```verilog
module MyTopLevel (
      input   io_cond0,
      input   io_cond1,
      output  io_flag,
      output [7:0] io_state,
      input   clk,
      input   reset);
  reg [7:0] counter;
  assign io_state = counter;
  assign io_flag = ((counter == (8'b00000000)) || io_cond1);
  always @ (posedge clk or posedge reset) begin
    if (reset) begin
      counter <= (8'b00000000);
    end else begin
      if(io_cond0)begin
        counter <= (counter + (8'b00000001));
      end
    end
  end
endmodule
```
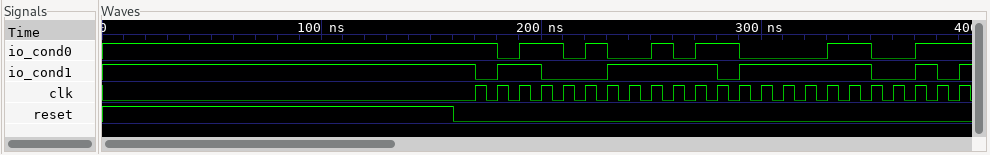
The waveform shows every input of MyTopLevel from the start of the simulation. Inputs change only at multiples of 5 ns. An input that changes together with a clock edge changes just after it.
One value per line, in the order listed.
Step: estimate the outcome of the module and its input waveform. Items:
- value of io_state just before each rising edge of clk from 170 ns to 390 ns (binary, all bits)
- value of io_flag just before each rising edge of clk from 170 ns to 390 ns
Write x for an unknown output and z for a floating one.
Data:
00000000, 00000001, 00000010, 00000010, 00000011, 00000100, 00000100, 00000101, 00000101, 00000101, 00000110, 00000110, 00000111, 00001000, 00001000, 00001000, 00001000, 00001000, 00001001, 00001010, 00001010, 00001010, 00001011
1 0 1 1 0 0 0 1 1 1 1 1 0 1 1 1 1 1 1 0 0 1 0
